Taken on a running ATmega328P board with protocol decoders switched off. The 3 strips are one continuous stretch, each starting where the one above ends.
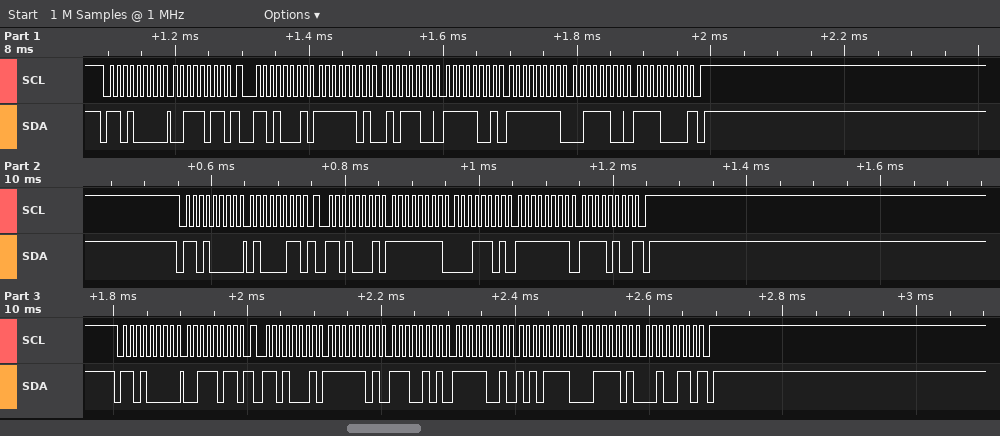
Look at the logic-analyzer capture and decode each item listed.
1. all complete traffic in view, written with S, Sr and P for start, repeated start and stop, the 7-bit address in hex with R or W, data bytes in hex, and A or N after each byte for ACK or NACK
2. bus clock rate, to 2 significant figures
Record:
S 68W A 3B A Sr 68R A FD A 5C A F9 A FF A 3C A F0 N P S 68W A 43 A Sr 68R A FF A 1D A FF A F4 N P S 68W A 3B A Sr 68R A FD A E5 A F9 A AF A 3D A 26 N P
100 kHz
